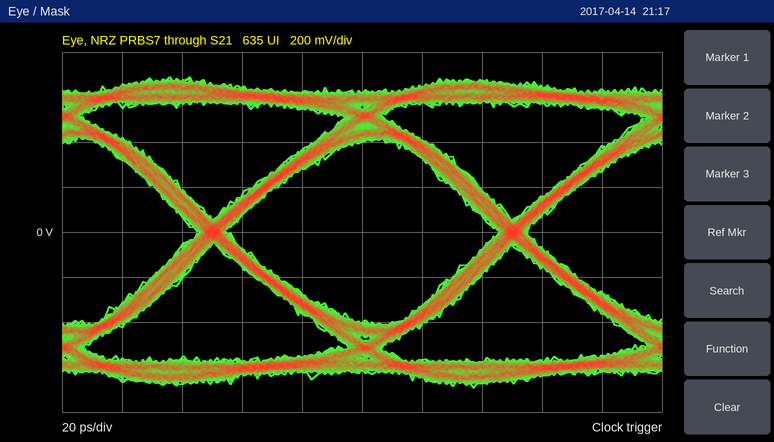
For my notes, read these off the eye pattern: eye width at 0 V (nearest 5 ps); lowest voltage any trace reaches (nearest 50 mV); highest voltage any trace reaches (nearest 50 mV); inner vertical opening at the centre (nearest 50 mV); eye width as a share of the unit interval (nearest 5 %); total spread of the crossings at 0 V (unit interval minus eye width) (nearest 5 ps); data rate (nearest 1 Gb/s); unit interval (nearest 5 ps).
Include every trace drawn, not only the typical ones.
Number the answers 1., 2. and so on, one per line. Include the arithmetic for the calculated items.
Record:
1. 90 ps
2. -700 mV
3. 700 mV
4. 800 mV
5. 90 ps / 100 ps ≈ 90 %
6. 10 ps
7. 10 Gb/s
8. 100 ps
